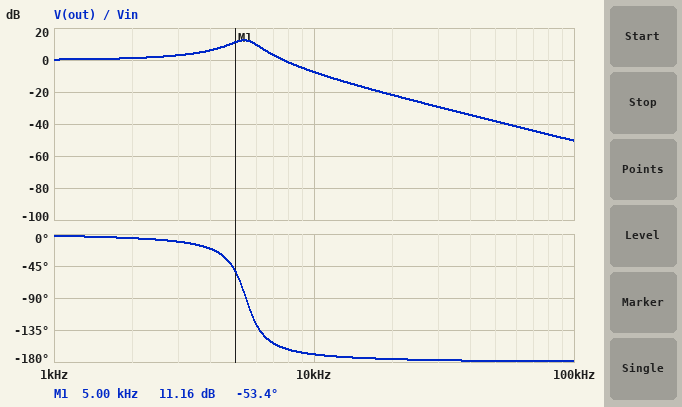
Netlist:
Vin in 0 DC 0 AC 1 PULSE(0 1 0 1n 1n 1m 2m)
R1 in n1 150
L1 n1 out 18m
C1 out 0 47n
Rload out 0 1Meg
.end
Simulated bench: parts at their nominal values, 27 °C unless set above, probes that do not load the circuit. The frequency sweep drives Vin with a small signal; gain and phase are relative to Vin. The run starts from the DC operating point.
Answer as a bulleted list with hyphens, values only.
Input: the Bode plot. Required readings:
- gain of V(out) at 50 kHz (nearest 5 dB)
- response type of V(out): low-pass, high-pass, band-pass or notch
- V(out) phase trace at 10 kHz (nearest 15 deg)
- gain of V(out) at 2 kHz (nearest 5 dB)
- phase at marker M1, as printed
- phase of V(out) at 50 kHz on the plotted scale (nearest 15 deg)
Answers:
- -40 dB
- low-pass
- -165 deg
- 0 dB
- -53.4 deg
- -180 deg
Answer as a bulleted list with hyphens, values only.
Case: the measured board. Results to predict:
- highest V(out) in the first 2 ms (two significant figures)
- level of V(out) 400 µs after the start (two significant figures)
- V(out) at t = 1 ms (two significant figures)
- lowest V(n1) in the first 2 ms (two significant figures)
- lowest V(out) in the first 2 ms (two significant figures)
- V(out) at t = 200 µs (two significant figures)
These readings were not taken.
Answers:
- 1.7 V
- 890 mV
- 1.0 V
- -140 mV
- -690 mV
- 600 mV
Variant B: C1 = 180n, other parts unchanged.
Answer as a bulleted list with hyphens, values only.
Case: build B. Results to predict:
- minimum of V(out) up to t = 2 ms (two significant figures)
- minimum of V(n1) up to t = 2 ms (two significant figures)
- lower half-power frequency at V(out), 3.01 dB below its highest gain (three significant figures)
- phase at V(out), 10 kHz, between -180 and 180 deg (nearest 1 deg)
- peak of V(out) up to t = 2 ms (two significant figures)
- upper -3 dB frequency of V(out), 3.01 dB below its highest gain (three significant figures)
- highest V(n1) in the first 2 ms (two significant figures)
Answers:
- -470 mV
- -160 mV
- 1.83 kHz
- -172 deg
- 1.5 V
- 3.25 kHz
- 1.2 V
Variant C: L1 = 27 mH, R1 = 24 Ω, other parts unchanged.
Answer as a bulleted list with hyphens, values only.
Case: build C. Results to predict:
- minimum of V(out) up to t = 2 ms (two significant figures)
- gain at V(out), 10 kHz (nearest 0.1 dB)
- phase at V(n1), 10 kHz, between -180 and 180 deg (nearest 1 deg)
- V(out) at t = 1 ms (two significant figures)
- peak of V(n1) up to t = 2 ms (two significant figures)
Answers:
- -1.5 V
- -12.1 dB
- 1 deg
- 1.6 V
- 1.0 V
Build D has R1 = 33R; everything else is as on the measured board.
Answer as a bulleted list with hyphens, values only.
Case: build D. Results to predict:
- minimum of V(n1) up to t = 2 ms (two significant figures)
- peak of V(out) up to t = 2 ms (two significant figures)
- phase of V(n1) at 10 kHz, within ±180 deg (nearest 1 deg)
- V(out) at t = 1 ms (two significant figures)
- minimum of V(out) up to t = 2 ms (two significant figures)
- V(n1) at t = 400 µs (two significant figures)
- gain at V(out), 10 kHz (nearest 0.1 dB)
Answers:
- -65 mV
- 1.9 V
- 2 deg
- 1.4 V
- -1.3 V
- 970 mV
- -7.4 dB
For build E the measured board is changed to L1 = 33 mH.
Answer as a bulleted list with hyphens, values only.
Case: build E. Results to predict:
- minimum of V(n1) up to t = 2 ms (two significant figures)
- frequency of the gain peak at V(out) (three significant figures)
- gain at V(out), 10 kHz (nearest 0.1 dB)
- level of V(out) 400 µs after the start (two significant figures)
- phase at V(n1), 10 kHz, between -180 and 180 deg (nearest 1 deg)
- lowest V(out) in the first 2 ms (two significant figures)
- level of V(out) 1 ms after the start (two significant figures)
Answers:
- -110 mV
- 4.01 kHz
- -14.2 dB
- 1.3 V
- 5 deg
- -680 mV
- 900 mV
